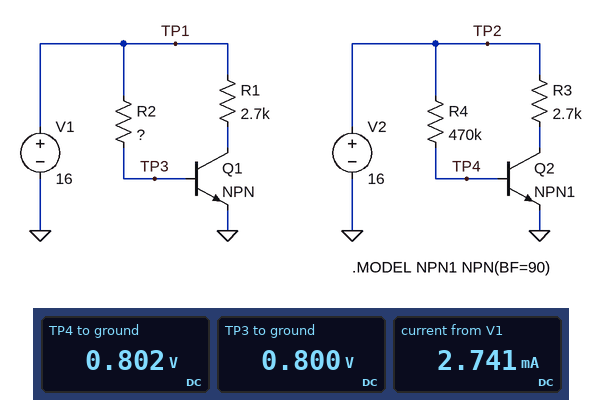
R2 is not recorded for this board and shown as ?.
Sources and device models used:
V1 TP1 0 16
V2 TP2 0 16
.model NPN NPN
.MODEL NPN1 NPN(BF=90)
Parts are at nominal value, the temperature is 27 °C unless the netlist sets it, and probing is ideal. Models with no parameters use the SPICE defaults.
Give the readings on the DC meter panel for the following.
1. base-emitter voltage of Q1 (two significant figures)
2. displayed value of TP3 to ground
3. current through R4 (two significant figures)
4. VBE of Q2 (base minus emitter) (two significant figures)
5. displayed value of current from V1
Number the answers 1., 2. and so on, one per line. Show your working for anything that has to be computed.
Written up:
1. 800 mV = 800 mV
2. 0.800 V
3. (16 V - 802 mV) / 470 kΩ = 32 µA
4. 802 mV = 800 mV
5. 2.741 mA
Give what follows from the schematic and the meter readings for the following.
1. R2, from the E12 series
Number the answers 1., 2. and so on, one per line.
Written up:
1. 560 kΩ
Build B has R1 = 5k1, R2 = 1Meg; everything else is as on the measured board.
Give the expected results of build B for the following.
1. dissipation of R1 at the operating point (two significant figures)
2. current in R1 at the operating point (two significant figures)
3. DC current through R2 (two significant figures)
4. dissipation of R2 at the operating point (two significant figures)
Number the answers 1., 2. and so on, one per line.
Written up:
1. 12 mW
2. 1.5 mA
3. 15 µA
4. 230 µW
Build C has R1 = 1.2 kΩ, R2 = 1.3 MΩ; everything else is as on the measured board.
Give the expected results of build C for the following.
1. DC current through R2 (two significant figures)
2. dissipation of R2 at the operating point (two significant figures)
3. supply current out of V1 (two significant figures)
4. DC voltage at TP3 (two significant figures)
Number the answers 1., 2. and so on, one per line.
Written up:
1. 12 µA
2. 180 µW
3. 1.2 mA
4. 780 mV
